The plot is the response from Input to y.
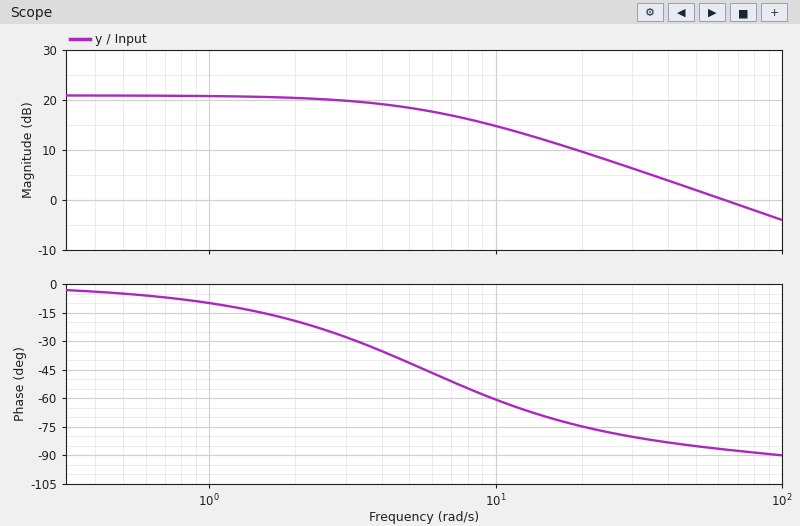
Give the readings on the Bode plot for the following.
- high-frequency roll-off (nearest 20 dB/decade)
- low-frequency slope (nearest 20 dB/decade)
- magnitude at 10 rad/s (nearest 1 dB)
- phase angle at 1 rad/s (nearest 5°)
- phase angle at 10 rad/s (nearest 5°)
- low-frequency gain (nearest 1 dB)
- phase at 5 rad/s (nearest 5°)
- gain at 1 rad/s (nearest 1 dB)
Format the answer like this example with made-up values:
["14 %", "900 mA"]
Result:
["-20 dB/decade", "0 dB/decade", "15 dB", "-10°", "-60°", "21 dB", "-40°", "21 dB"]
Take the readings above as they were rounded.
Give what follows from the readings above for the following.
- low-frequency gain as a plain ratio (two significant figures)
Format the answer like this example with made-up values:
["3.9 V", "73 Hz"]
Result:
["11"]
